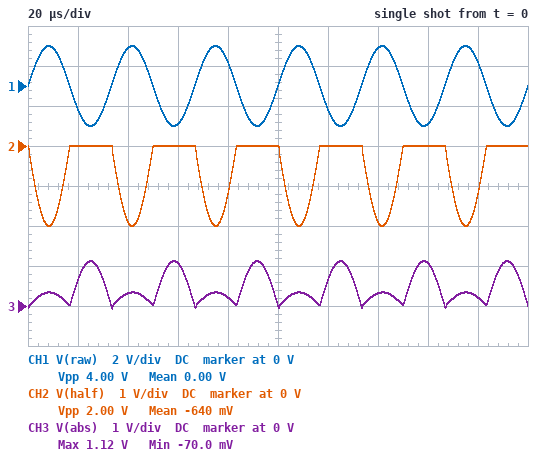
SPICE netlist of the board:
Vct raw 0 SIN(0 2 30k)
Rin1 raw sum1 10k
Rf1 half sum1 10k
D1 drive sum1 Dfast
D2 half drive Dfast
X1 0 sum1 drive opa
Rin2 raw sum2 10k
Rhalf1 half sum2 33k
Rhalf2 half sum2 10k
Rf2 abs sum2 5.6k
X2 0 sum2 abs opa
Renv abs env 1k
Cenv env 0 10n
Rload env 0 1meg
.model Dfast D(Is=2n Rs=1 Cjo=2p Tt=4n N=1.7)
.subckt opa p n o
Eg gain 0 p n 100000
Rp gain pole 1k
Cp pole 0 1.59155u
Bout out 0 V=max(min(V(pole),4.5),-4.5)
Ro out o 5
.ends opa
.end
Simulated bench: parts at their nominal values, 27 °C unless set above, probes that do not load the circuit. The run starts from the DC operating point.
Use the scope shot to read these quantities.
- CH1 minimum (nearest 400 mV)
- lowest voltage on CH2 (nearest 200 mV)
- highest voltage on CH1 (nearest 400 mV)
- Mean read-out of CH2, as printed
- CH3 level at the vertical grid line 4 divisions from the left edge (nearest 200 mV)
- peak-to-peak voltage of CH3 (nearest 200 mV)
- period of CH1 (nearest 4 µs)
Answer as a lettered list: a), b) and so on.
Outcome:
a) -2.0 V
b) -2.0 V
c) 2.0 V
d) -640 mV
e) 200 mV
f) 1.2 V
g) 32 µs
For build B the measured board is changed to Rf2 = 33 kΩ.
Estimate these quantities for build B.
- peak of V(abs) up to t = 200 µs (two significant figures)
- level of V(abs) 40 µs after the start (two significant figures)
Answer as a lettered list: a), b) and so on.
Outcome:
a) 4.5 V
b) 1.9 V
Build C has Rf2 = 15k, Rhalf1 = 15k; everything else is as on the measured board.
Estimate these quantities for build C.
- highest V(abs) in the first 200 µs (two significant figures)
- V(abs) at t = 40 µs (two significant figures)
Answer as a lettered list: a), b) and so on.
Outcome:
a) 3.0 V
b) 1.9 V
